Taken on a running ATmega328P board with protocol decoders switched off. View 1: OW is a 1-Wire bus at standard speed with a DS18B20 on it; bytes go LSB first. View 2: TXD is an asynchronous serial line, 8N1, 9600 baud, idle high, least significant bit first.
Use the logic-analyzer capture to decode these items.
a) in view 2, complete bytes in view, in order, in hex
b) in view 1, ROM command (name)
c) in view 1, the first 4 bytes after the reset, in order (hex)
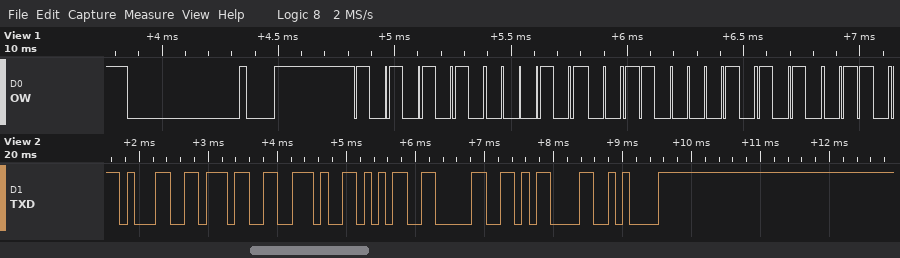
31 37 2E 35 30 0D 0A
Match ROM
55 28 43 65
